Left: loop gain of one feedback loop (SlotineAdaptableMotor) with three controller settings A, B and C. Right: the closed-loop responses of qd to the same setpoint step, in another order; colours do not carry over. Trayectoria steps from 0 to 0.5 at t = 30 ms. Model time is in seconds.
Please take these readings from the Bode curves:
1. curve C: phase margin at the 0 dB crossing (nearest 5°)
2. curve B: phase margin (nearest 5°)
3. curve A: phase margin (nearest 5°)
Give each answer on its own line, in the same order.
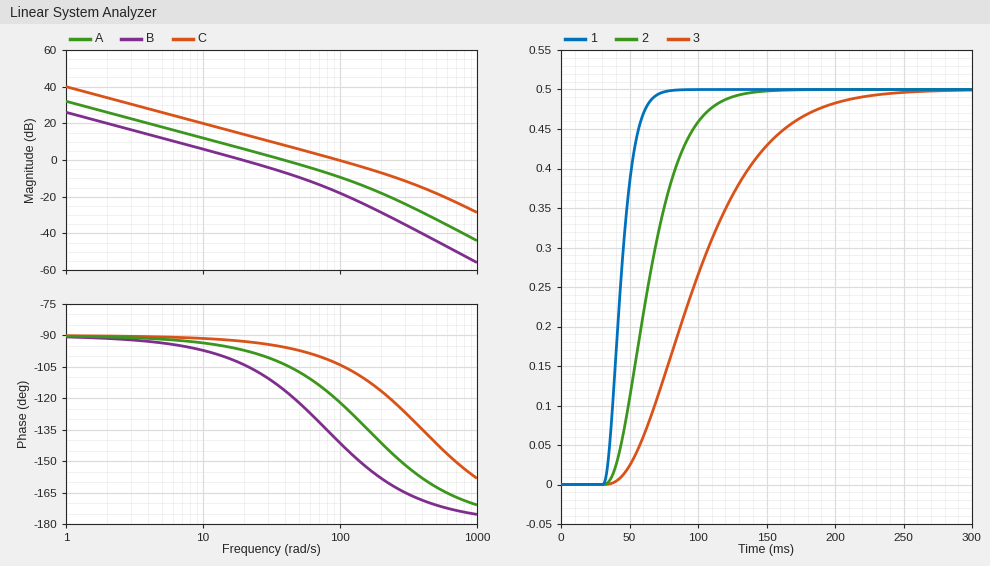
75°
75°
75°
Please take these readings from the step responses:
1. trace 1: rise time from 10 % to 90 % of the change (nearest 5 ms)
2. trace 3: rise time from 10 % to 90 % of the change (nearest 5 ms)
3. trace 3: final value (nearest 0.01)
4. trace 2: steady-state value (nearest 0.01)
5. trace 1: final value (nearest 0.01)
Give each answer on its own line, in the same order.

20 ms
105 ms
0.50
0.50
0.50
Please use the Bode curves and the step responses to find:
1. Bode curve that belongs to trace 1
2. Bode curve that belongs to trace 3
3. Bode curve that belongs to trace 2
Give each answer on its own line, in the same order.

C
B
A
